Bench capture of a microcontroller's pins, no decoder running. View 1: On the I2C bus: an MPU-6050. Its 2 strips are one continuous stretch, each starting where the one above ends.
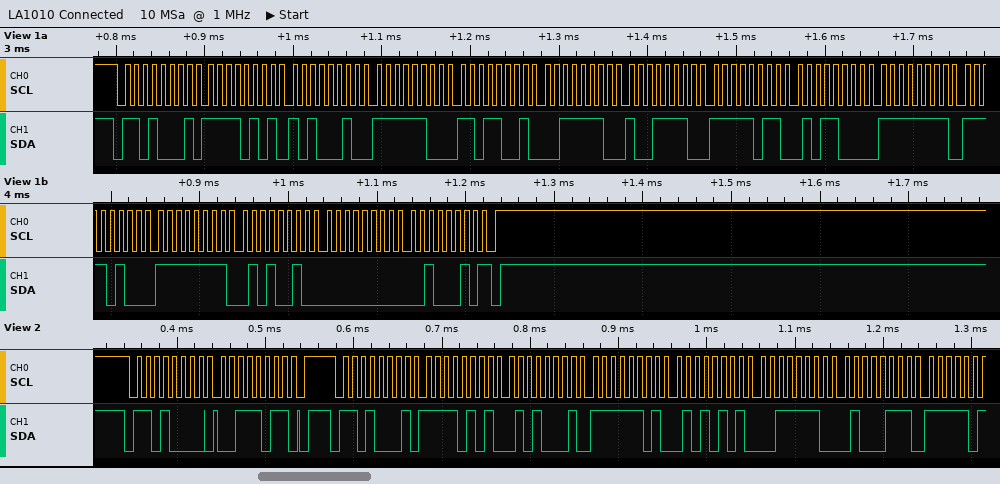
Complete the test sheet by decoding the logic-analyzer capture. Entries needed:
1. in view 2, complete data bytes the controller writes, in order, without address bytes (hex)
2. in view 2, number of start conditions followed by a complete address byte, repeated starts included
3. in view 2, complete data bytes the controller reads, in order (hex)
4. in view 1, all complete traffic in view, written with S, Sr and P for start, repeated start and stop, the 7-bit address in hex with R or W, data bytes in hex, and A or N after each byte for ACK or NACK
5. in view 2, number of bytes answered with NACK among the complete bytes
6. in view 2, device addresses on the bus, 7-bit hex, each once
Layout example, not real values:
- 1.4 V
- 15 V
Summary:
- 3B
- 2
- F5 51 FD 55 3E 47
- S 68R A F5 A A2 A FC A D9 A 3E A 9E A FB A 58 A FF A F4 A FF A 52 A 00 A 22 N P
- 0
- 0x68
